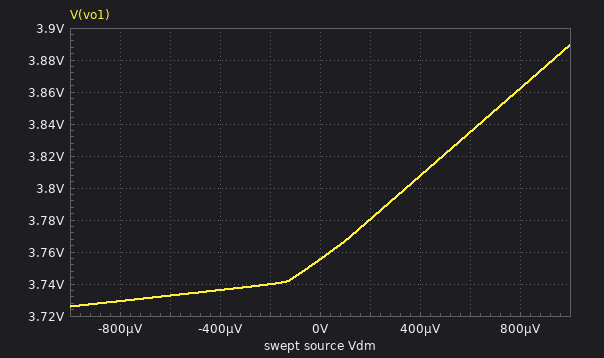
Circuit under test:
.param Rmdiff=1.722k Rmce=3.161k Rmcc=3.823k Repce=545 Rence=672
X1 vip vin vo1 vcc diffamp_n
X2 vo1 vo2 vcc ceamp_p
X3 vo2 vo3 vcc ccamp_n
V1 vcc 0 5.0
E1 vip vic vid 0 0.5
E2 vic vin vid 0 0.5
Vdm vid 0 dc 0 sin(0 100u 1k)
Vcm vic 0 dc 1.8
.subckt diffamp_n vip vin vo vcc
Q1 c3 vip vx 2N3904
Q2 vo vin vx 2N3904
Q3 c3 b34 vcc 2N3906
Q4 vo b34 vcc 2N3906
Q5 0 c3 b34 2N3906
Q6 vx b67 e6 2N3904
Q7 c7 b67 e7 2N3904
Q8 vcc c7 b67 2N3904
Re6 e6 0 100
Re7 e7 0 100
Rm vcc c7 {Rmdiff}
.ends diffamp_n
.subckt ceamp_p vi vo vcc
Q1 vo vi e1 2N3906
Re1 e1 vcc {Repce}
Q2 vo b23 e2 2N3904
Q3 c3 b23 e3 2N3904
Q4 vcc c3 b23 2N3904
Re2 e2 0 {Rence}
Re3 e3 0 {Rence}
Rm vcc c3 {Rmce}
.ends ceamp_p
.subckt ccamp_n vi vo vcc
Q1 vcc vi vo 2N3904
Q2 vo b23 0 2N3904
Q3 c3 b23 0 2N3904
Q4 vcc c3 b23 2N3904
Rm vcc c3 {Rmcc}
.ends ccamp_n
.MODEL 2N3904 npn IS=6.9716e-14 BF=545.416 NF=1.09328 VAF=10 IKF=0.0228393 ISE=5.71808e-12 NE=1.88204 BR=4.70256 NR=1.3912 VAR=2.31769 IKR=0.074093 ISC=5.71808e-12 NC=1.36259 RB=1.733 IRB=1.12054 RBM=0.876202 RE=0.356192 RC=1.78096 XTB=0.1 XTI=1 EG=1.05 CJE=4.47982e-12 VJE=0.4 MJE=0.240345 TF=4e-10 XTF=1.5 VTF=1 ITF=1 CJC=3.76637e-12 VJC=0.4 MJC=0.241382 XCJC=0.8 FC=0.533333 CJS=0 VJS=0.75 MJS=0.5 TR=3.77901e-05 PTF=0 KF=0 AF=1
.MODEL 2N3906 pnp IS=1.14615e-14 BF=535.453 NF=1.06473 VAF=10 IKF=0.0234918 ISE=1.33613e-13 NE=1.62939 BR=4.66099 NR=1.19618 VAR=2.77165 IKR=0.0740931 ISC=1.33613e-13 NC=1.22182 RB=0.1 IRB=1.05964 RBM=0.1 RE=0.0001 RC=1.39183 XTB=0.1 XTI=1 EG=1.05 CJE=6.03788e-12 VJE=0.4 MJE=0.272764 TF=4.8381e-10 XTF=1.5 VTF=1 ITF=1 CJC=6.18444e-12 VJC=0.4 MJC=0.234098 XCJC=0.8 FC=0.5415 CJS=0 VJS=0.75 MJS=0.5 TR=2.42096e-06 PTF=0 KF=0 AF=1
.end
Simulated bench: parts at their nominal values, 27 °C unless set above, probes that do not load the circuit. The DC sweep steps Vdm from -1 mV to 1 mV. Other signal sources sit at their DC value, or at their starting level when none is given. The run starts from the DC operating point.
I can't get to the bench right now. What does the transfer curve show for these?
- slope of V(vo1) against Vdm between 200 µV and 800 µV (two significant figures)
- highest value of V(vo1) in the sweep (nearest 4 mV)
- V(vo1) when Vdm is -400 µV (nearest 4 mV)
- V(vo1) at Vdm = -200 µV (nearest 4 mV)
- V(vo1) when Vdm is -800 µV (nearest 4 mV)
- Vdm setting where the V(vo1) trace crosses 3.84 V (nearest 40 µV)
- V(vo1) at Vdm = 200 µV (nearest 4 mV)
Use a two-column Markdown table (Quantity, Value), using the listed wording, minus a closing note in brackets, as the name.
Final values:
| Quantity | Value |
|---|---|
| slope of V(vo1) against Vdm between 200 µV and 800 µV | 140 V/V |
| highest value of V(vo1) in the sweep | 3.888 V |
| V(vo1) when Vdm is -400 µV | 3.736 V |
| V(vo1) at Vdm = -200 µV | 3.740 V |
| V(vo1) when Vdm is -800 µV | 3.728 V |
| Vdm setting where the V(vo1) trace crosses 3.84 V | 640 µV |
| V(vo1) at Vdm = 200 µV | 3.780 V |
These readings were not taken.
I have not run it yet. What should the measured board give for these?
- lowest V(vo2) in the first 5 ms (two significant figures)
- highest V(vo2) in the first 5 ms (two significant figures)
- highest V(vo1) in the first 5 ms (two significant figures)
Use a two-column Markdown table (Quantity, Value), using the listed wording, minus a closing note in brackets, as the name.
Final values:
| Quantity | Value |
|---|---|
| lowest V(vo2) in the first 5 ms | 1.0 V |
| highest V(vo2) in the first 5 ms | 3.8 V |
| highest V(vo1) in the first 5 ms | 3.8 V |
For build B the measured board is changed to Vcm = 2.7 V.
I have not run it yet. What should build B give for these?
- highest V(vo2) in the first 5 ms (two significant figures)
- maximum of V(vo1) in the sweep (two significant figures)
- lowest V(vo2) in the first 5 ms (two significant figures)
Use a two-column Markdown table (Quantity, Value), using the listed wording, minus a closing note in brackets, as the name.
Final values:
| Quantity | Value |
|---|---|
| highest V(vo2) in the first 5 ms | 4.0 V |
| maximum of V(vo1) in the sweep | 3.9 V |
| lowest V(vo2) in the first 5 ms | 1.3 V |
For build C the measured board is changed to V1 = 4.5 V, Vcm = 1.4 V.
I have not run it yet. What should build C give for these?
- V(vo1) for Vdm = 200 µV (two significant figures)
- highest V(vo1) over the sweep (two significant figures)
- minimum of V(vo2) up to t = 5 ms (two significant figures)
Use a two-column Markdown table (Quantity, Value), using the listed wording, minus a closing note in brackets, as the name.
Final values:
| Quantity | Value |
|---|---|
| V(vo1) for Vdm = 200 µV | 3.3 V |
| highest V(vo1) over the sweep | 3.4 V |
| minimum of V(vo2) up to t = 5 ms | 3.9 V |
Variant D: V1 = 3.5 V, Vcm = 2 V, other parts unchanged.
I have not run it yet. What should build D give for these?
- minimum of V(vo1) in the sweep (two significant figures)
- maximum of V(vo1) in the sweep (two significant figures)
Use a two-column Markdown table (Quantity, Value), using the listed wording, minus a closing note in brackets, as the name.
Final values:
| Quantity | Value |
|---|---|
| minimum of V(vo1) in the sweep | 2.4 V |
| maximum of V(vo1) in the sweep | 2.5 V |
